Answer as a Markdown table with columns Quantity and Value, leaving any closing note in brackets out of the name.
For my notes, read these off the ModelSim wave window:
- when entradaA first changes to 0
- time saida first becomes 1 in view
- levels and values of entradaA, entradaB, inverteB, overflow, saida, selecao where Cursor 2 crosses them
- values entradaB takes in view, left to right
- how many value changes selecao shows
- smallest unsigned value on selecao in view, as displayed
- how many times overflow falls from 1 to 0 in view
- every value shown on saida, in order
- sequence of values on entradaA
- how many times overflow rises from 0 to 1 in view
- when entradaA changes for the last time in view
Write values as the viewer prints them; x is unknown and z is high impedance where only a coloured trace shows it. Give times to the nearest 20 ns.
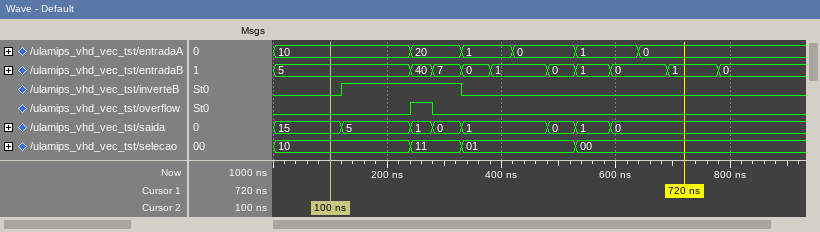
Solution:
| Quantity | Value |
|---|---|
| when entradaA first changes to 0 | 420 ns |
| time saida first becomes 1 in view | 240 ns |
| levels and values of entradaA, entradaB, inverteB, overflow, saida, selecao where Cursor 2 crosses them | entradaA=10, entradaB=5, inverteB=0, overflow=0, saida=15, selecao=10 |
| values entradaB takes in view, left to right | 5, 40, 7, 0, 1, 0, 1, 0, 1, 0 |
| how many value changes selecao shows | 3 |
| smallest unsigned value on selecao in view, as displayed | 00 |
| how many times overflow falls from 1 to 0 in view | 1 |
| every value shown on saida, in order | 15, 5, 1, 0, 1, 0, 1, 0 |
| sequence of values on entradaA | 10, 20, 1, 0, 1, 0 |
| how many times overflow rises from 0 to 1 in view | 1 |
| when entradaA changes for the last time in view | 640 ns |
